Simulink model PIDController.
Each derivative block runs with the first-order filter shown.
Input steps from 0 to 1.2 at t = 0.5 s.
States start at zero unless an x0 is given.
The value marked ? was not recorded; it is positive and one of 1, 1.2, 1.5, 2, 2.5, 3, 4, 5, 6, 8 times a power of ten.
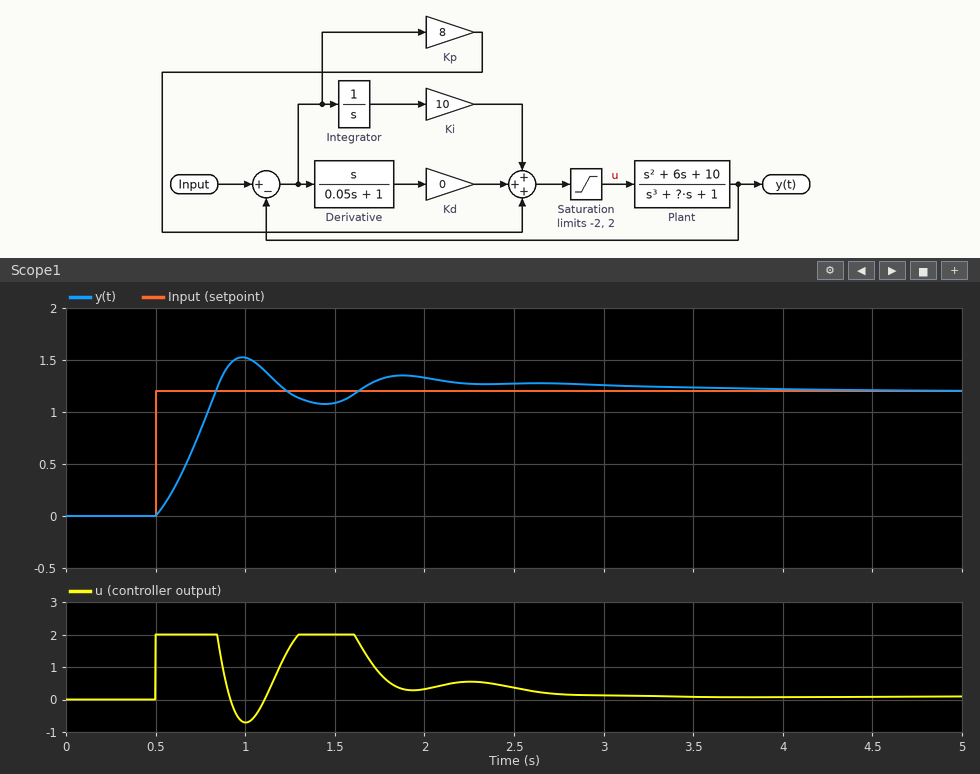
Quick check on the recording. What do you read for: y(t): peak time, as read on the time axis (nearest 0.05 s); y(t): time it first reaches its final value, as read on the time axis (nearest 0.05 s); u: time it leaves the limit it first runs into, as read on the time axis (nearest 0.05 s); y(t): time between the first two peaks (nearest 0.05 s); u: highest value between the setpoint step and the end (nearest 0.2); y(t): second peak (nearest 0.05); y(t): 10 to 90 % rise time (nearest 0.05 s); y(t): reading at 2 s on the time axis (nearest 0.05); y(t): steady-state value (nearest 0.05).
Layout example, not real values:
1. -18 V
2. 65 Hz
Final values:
1. 1.00 s
2. 0.85 s
3. 0.85 s
4. 0.90 s
5. 2.0
6. 1.35
7. 0.25 s
8. 1.35
9. 1.20
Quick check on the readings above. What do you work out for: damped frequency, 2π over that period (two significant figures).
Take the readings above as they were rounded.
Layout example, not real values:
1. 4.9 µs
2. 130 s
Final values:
1. 7.0 rad/s
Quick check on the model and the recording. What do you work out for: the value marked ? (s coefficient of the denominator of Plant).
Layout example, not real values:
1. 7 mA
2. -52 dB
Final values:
1. 15
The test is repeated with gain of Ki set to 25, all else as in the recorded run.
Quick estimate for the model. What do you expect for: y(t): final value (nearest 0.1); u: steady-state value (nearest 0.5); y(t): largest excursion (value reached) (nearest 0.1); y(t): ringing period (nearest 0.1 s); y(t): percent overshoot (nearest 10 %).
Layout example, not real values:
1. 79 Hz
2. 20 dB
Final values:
1. 1.2
2. 0.0
3. 1.8
4. 1.0 s
5. 50 %
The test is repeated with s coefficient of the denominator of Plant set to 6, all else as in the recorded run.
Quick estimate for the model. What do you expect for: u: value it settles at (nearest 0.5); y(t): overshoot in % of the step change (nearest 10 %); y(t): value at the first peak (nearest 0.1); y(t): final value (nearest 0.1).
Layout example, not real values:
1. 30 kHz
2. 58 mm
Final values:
1. 0.0
2. 40 %
3. 1.7
4. 1.2
